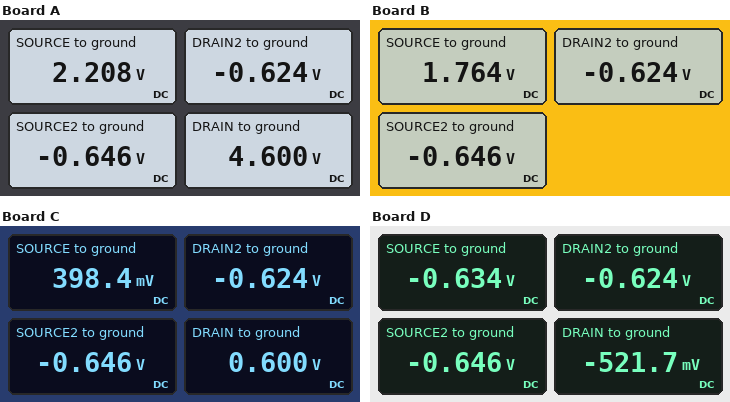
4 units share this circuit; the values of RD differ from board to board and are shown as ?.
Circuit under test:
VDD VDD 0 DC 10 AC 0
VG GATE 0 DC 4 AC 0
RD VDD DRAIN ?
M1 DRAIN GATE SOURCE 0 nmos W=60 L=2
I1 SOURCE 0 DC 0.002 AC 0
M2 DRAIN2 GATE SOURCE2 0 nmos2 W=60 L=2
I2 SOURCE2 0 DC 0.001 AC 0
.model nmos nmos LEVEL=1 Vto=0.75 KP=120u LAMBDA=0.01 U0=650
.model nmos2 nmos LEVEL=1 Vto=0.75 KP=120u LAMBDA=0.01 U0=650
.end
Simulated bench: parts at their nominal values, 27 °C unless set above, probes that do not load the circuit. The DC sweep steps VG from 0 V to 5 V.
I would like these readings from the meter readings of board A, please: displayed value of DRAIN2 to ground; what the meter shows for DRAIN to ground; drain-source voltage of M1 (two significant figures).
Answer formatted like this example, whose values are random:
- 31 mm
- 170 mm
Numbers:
- -0.624 V
- 4.600 V
- 2.4 V
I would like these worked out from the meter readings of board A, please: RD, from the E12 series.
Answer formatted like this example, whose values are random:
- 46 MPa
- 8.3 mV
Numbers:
- 2.7 kΩ
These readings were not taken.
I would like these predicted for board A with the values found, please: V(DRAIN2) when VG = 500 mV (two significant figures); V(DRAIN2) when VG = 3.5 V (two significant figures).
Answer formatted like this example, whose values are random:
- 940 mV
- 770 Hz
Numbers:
- -590 mV
- -620 mV
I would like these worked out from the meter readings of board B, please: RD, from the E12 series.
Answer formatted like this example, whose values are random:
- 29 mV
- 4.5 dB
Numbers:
- 3.9 kΩ
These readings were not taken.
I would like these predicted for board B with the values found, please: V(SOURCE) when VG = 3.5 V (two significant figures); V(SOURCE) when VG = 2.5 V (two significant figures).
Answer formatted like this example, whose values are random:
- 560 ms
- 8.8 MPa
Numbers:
- 1.6 V
- 700 mV
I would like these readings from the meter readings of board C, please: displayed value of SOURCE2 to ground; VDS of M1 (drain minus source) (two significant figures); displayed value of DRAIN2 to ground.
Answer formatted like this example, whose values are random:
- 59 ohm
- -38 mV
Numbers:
- -0.646 V
- 200 mV
- -0.624 V
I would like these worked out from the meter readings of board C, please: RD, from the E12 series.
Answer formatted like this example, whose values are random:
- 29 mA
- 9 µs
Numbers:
- 4.7 kΩ
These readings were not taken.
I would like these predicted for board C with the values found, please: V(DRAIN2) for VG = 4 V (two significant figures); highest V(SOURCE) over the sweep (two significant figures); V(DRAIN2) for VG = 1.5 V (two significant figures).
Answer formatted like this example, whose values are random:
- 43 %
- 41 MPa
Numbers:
- -620 mV
- 450 mV
- -610 mV
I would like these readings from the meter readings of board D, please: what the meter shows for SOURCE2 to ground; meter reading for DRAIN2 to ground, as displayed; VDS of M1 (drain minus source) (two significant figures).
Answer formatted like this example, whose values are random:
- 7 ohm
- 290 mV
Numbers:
- -0.646 V
- -0.624 V
- 110 mV
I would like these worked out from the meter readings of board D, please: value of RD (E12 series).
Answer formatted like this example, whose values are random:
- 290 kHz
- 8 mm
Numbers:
- 6.8 kΩ
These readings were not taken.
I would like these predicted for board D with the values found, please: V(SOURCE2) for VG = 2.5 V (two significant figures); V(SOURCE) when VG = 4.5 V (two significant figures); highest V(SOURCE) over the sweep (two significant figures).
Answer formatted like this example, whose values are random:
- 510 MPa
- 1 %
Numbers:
- -650 mV
- -630 mV
- -630 mV
